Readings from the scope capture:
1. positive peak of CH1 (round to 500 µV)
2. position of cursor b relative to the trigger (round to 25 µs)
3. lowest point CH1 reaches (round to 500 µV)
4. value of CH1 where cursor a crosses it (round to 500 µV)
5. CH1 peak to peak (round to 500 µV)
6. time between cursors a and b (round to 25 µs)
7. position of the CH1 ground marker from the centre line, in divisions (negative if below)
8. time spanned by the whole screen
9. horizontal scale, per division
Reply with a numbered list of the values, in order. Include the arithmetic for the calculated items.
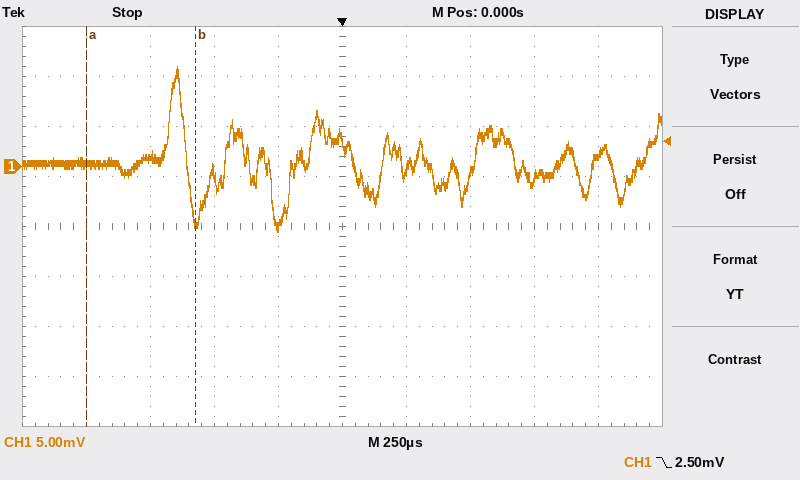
1. 10.0 mV
2. -575 µs
3. -6.5 mV
4. 0.0 mV
5. 10.0 mV − (-6.5 mV) = 16.5 mV
6. 425 µs
7. +1.2 div
8. 2.5 ms
9. 250 µs
